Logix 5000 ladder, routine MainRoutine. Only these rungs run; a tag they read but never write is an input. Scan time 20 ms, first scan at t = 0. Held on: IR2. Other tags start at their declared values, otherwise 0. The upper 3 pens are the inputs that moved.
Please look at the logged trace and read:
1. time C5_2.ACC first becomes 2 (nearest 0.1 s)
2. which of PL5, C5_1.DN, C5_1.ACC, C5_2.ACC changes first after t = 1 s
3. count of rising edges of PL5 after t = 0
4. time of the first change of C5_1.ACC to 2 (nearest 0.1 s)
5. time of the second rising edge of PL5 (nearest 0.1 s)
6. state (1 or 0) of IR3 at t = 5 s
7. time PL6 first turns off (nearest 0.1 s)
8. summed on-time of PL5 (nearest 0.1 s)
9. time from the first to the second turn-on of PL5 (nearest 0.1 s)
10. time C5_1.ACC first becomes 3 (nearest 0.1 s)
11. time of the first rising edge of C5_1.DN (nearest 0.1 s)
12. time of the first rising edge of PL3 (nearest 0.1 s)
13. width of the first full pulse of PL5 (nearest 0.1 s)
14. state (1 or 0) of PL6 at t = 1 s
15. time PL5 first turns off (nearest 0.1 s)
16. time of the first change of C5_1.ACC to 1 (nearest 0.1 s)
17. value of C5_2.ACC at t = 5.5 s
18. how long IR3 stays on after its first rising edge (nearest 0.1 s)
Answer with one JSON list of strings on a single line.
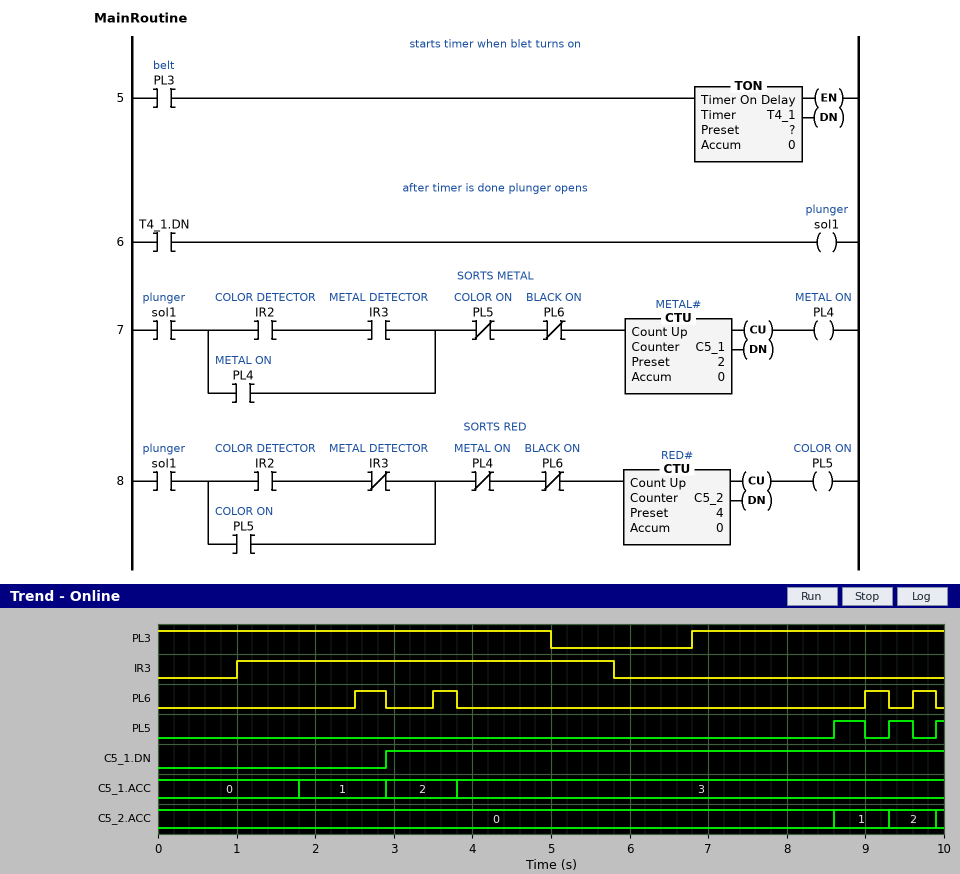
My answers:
["9.3 s", "C5_1.ACC", "3", "2.9 s", "9.3 s", "1", "2.9 s", "0.8 s", "0.7 s", "3.8 s", "2.9 s", "6.8 s", "0.4 s", "0", "9.0 s", "1.8 s", "0", "4.8 s"]
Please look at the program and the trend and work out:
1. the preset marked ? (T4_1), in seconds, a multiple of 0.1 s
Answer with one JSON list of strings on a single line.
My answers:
["1.8 s"]
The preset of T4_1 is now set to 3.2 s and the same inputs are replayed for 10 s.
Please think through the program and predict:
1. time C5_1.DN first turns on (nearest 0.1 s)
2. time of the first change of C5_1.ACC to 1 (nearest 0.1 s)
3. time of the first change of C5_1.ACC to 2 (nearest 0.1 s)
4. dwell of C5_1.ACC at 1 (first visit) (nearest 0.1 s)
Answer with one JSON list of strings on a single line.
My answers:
["3.8 s", "3.2 s", "3.8 s", "0.6 s"]
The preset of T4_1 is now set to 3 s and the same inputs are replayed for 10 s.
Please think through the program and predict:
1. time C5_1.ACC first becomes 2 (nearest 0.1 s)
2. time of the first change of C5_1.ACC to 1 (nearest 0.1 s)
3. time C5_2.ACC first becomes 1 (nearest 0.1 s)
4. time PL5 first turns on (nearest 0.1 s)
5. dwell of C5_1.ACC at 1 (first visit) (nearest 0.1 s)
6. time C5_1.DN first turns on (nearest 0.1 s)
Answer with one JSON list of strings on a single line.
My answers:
["3.8 s", "3.0 s", "9.9 s", "9.9 s", "0.8 s", "3.8 s"]
